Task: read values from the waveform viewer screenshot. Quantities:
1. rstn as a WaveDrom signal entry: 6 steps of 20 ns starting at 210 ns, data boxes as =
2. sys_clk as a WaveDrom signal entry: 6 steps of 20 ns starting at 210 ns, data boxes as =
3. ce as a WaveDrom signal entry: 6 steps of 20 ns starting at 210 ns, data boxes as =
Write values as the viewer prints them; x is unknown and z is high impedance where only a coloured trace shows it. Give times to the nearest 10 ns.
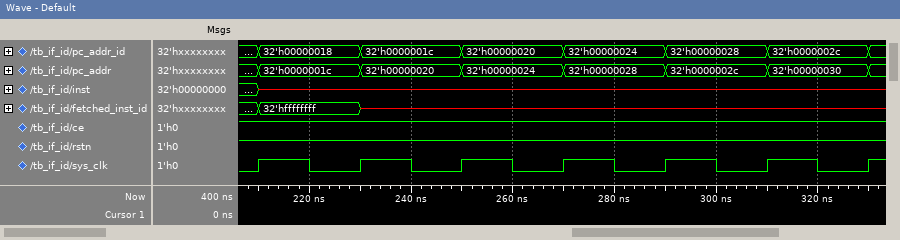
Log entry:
{name: 'rstn', wave: '1.....'}
{name: 'sys_clk', wave: 'p.....'}
{name: 'ce', wave: '1.....'}
